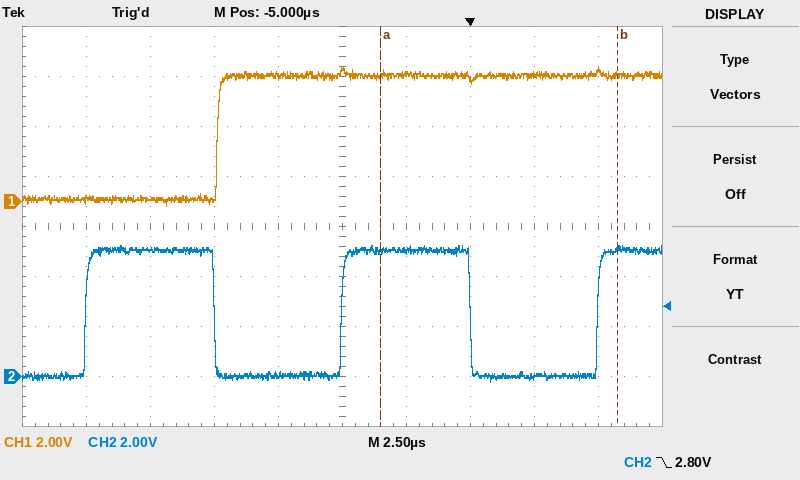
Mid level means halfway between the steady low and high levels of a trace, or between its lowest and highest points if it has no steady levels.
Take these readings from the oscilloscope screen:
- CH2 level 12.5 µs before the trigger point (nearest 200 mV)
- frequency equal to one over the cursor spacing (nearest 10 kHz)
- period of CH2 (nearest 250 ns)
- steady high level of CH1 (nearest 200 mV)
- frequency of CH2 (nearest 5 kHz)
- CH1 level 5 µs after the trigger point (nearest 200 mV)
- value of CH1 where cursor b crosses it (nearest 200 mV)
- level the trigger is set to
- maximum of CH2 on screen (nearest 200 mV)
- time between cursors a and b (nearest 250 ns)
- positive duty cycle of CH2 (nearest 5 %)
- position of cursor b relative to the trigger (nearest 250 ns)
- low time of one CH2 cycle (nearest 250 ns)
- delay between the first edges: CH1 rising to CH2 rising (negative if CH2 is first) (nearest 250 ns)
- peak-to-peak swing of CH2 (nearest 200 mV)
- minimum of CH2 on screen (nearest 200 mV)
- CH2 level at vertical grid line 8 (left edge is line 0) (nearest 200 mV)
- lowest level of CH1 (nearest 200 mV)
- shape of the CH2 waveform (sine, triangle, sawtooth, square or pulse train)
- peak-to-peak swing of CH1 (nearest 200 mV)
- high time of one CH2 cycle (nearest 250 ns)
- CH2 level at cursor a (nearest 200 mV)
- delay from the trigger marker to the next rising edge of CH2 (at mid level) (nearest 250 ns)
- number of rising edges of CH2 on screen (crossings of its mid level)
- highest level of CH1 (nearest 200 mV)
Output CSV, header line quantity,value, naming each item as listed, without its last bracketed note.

quantity,value
CH2 level 12.5 µs before the trigger point,5.0 V
frequency equal to one over the cursor spacing,110 kHz
period of CH2,10.00 µs
steady high level of CH1,5.0 V
frequency of CH2,100 kHz
CH1 level 5 µs after the trigger point,5.2 V
value of CH1 where cursor b crosses it,5.0 V
level the trigger is set to,2.80 V
maximum of CH2 on screen,5.2 V
time between cursors a and b,9.25 µs
positive duty cycle of CH2,50 %
position of cursor b relative to the trigger,+5.75 µs
low time of one CH2 cycle,5.00 µs
delay between the first edges: CH1 rising to CH2 rising (negative if CH2 is first),-5.25 µs
peak-to-peak swing of CH2,5.4 V
minimum of CH2 on screen,-200 mV
CH2 level at vertical grid line 8 (left edge is line 0),0.0 V
lowest level of CH1,-200 mV
shape of the CH2 waveform,square
peak-to-peak swing of CH1,5.6 V
high time of one CH2 cycle,5.00 µs
CH2 level at cursor a,5.0 V
delay from the trigger marker to the next rising edge of CH2 (at mid level),5.00 µs
number of rising edges of CH2 on screen,3
highest level of CH1,5.4 V
